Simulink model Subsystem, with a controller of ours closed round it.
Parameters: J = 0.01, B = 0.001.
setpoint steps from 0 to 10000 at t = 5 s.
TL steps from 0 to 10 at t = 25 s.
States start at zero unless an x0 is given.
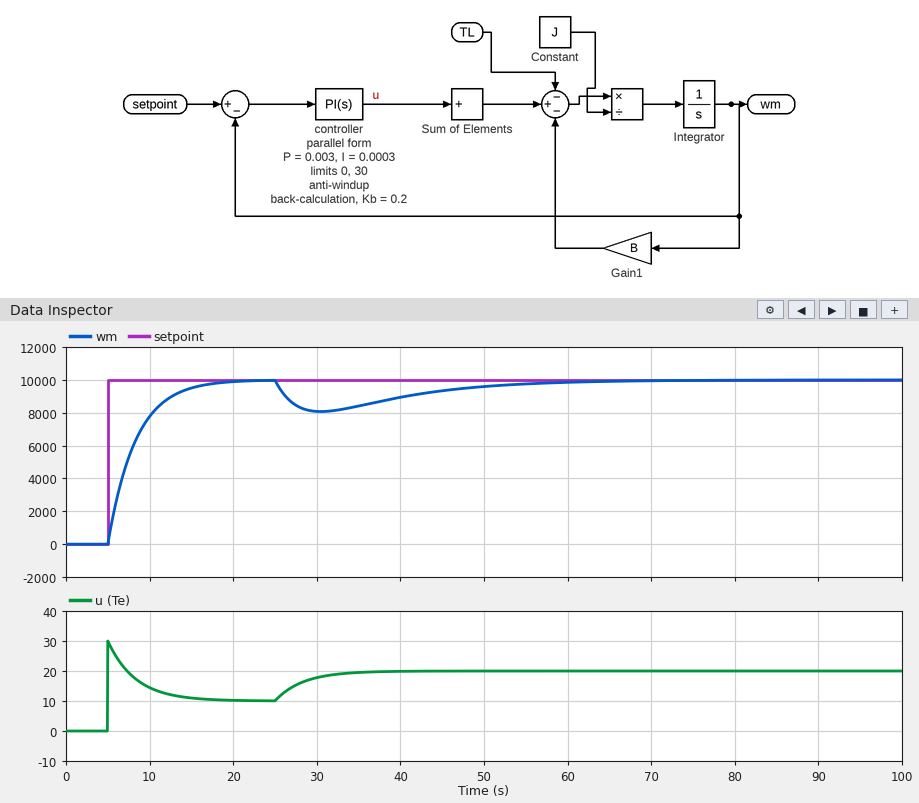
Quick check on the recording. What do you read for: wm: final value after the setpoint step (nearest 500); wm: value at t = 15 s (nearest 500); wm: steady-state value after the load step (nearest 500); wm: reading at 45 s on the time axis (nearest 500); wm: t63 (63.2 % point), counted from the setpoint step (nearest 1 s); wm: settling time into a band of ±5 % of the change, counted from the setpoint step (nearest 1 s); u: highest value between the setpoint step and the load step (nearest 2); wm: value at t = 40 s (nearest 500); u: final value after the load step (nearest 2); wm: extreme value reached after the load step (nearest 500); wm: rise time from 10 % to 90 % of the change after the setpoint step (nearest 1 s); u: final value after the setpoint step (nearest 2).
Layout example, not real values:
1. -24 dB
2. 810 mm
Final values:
1. 10000
2. 9500
3. 10000
4. 9500
5. 3 s
6. 10 s
7. 30
8. 9000
9. 20
10. 8000
11. 7 s
12. 10
